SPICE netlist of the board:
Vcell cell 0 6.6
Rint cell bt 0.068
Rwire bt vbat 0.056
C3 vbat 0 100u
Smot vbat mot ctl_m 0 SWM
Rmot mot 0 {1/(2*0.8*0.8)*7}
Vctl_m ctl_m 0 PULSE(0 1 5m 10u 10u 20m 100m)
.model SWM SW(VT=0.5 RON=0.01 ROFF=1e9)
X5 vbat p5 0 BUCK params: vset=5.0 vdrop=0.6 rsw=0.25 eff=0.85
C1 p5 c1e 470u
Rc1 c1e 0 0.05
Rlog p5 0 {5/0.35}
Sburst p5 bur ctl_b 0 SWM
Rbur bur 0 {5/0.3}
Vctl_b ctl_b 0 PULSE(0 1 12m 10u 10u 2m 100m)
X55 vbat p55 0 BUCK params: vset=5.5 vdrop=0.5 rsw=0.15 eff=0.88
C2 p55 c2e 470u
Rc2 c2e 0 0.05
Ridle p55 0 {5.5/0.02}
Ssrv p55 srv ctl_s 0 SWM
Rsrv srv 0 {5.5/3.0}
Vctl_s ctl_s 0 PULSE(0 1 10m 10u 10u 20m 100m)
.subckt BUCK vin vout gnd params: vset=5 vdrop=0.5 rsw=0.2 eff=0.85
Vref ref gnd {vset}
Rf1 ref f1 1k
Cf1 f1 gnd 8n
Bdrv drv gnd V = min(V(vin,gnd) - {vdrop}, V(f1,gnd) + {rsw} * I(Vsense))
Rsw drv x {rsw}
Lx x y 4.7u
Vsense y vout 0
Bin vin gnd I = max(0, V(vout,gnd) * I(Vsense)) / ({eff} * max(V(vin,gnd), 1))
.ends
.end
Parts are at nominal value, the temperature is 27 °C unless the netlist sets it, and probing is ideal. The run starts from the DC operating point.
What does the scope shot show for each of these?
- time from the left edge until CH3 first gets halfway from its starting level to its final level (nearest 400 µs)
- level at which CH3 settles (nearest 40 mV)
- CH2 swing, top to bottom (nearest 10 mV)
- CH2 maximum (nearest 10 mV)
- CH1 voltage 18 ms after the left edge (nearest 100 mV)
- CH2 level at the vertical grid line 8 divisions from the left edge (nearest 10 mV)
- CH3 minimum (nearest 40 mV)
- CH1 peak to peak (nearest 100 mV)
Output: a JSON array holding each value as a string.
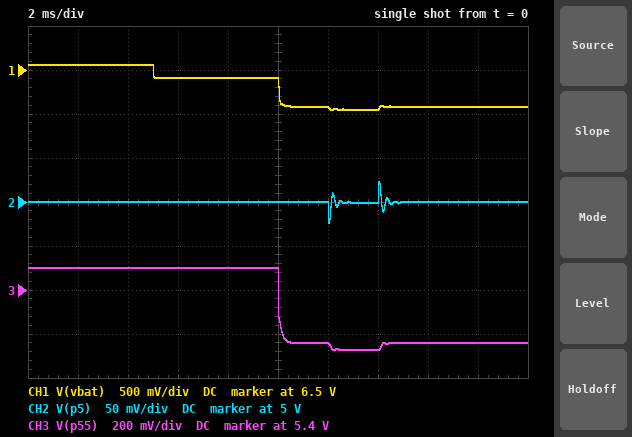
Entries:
["10.0 ms", "5.16 V", "50 mV", "5.02 V", "6.1 V", "5.00 V", "5.12 V", "500 mV"]
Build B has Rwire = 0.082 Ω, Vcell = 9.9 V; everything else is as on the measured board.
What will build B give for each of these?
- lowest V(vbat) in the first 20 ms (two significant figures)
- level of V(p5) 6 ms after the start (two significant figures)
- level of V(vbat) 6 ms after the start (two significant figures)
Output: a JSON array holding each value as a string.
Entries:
["9.2 V", "5.0 V", "9.6 V"]
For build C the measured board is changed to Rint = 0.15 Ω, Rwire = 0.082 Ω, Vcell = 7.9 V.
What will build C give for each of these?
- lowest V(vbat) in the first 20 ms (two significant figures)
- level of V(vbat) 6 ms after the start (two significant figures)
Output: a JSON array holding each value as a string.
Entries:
["6.6 V", "7.5 V"]
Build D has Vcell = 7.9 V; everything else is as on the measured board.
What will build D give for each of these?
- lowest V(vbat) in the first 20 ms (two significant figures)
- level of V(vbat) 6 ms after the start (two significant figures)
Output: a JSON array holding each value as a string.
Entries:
["7.2 V", "7.7 V"]
